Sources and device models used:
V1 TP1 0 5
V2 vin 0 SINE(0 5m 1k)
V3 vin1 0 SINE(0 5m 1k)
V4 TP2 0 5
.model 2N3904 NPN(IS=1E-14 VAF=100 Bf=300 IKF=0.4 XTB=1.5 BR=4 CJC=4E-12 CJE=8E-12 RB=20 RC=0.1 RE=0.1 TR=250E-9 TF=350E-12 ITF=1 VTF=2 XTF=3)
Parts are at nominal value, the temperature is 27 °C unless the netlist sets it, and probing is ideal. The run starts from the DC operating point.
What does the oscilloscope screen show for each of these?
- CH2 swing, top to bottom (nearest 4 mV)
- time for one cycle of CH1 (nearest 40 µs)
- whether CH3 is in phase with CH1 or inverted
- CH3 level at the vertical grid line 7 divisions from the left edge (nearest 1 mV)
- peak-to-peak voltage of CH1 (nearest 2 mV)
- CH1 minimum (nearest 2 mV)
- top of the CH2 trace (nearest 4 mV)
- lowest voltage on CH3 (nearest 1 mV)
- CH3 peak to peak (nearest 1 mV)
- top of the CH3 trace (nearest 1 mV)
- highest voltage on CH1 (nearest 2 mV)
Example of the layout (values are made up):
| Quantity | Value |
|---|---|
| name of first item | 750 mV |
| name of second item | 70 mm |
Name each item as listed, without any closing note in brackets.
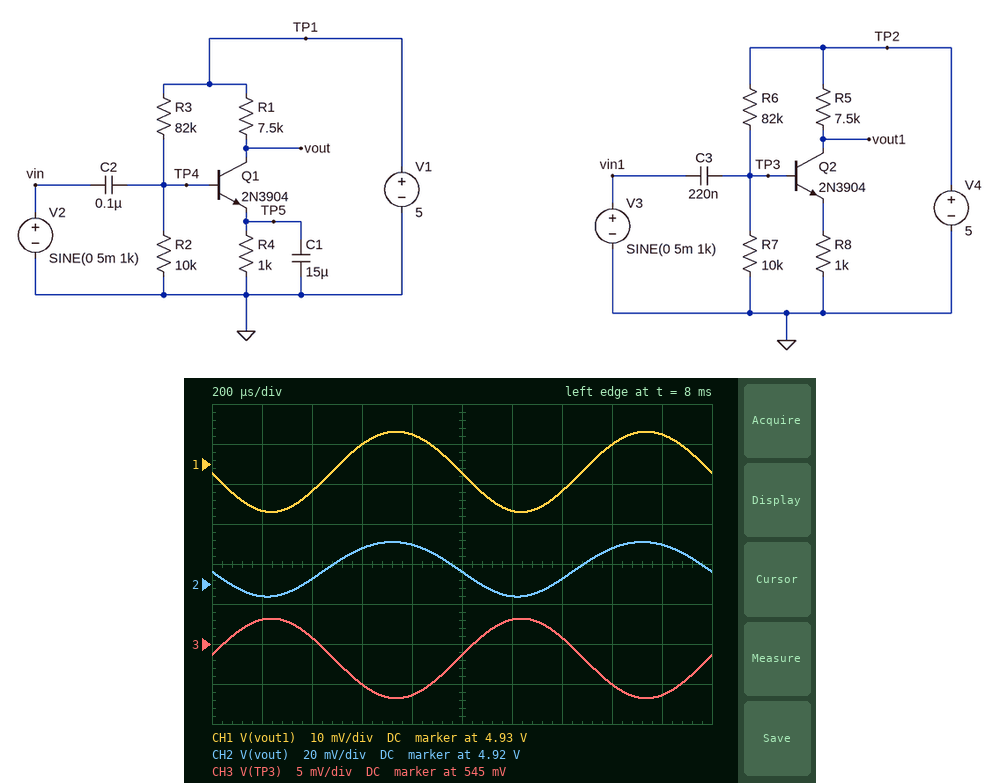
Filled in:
| Quantity | Value |
|---|---|
| CH2 swing, top to bottom | 28 mV |
| time for one cycle of CH1 | 1.00 ms |
| whether CH3 is in phase with CH1 or inverted | inverted |
| CH3 level at the vertical grid line 7 divisions from the left edge | 546 mV |
| peak-to-peak voltage of CH1 | 20 mV |
| CH1 minimum | 4.918 V |
| top of the CH2 trace | 4.940 V |
| lowest voltage on CH3 | 538 mV |
| CH3 peak to peak | 10 mV |
| top of the CH3 trace | 548 mV |
| highest voltage on CH1 | 4.938 V |
